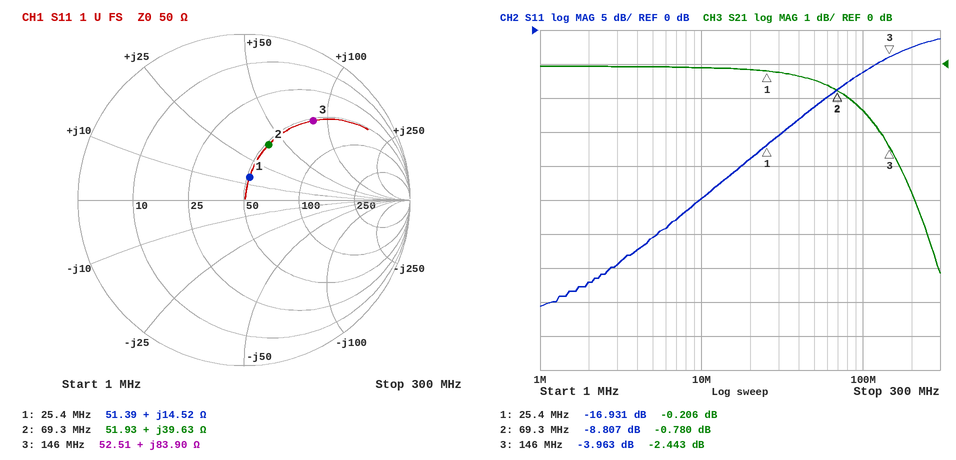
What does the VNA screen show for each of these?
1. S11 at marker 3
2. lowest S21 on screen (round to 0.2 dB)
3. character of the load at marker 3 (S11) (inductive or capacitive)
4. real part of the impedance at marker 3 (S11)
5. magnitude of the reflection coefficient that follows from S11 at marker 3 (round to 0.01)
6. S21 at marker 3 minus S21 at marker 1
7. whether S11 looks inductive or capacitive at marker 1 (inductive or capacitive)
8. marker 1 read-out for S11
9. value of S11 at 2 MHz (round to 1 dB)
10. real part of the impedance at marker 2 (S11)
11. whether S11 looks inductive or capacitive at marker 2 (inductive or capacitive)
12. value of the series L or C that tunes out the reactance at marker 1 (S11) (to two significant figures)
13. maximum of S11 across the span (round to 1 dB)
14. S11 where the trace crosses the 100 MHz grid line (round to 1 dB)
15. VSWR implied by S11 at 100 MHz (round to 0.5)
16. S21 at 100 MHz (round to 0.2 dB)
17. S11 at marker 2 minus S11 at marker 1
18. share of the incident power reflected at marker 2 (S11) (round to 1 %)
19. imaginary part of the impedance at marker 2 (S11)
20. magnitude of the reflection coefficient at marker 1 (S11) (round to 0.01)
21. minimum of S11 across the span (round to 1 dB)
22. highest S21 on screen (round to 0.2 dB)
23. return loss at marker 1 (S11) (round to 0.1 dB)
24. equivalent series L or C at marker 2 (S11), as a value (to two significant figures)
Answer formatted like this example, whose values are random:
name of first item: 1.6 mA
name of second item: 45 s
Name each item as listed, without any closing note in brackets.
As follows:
S11 at marker 3: -3.963 dB
lowest S21 on screen: -6.2 dB
character of the load at marker 3 (S11): inductive
real part of the impedance at marker 3: 52.51 Ω
magnitude of the reflection coefficient that follows from S11 at marker 3: 0.63
S21 at marker 3 minus S21 at marker 1: -2.237 dB
whether S11 looks inductive or capacitive at marker 1: inductive
marker 1 read-out for S11: -16.931 dB
value of S11 at 2 MHz: -37 dB
real part of the impedance at marker 2: 51.93 Ω
whether S11 looks inductive or capacitive at marker 2: inductive
value of the series L or C that tunes out the reactance at marker 1 (S11): 430 pF
maximum of S11 across the span: -1 dB
S11 where the trace crosses the 100 MHz grid line: -6 dB
VSWR implied by S11 at 100 MHz: 3.0
S21 at 100 MHz: -1.4 dB
S11 at marker 2 minus S11 at marker 1: 8.124 dB
share of the incident power reflected at marker 2 (S11): 13 %
imaginary part of the impedance at marker 2: +39.63 Ω
magnitude of the reflection coefficient at marker 1 (S11): 0.14
minimum of S11 across the span: -41 dB
highest S21 on screen: 0.0 dB
return loss at marker 1 (S11): 16.9 dB
equivalent series L or C at marker 2 (S11), as a value: 91 nH
